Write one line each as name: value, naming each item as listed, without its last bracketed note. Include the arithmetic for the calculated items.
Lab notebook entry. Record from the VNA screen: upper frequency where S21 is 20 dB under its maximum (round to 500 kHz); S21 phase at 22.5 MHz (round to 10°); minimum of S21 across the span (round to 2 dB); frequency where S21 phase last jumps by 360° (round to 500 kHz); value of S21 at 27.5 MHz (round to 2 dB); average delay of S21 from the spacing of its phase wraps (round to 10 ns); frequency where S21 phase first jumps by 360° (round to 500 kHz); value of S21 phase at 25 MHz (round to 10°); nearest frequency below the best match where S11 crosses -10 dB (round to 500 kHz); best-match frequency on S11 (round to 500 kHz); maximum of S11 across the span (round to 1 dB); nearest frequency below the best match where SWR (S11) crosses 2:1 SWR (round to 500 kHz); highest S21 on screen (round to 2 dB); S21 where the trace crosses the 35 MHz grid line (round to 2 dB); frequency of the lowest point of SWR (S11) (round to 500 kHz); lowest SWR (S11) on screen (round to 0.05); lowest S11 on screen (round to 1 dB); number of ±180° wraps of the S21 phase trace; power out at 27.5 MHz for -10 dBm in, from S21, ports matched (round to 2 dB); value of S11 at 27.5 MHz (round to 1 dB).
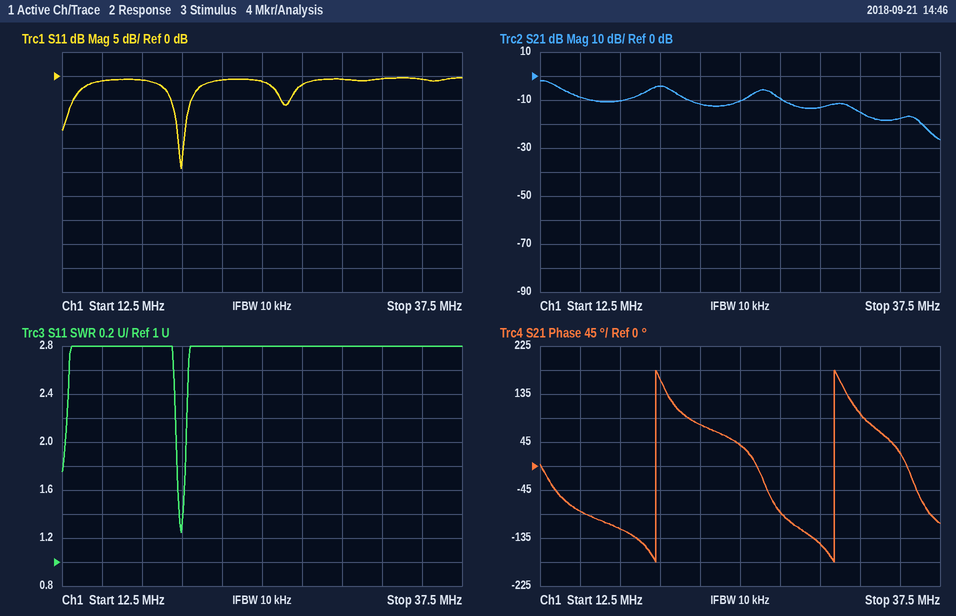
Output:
upper frequency where S21 is 20 dB under its maximum: 36.5 MHz
S21 phase at 22.5 MHz: 80°
minimum of S21 across the span: -26 dB
frequency where S21 phase last jumps by 360°: 31.0 MHz
value of S21 at 27.5 MHz: -10 dB
average delay of S21 from the spacing of its phase wraps: 1 cycle / (31.0 MHz − 19.5 MHz) ≈ 87.0 ns, so 90 ns to the nearest 10 ns
frequency where S21 phase first jumps by 360°: 19.5 MHz
value of S21 phase at 25 MHz: 40°
nearest frequency below the best match where S11 crosses -10 dB: 19.5 MHz
best-match frequency on S11: 20.0 MHz
maximum of S11 across the span: 0 dB
nearest frequency below the best match where SWR (S11) crosses 2:1 SWR: 19.5 MHz
highest S21 on screen: -2 dB
S21 where the trace crosses the 35 MHz grid line: -18 dB
frequency of the lowest point of SWR (S11): 20.0 MHz
lowest SWR (S11) on screen: 1.25
lowest S11 on screen: -19 dB
number of ±180° wraps of the S21 phase trace: 2
power out at 27.5 MHz for -10 dBm in, from S21, ports matched: -10 dBm + (-10 dB) = -20 dBm
value of S11 at 27.5 MHz: -2 dB
